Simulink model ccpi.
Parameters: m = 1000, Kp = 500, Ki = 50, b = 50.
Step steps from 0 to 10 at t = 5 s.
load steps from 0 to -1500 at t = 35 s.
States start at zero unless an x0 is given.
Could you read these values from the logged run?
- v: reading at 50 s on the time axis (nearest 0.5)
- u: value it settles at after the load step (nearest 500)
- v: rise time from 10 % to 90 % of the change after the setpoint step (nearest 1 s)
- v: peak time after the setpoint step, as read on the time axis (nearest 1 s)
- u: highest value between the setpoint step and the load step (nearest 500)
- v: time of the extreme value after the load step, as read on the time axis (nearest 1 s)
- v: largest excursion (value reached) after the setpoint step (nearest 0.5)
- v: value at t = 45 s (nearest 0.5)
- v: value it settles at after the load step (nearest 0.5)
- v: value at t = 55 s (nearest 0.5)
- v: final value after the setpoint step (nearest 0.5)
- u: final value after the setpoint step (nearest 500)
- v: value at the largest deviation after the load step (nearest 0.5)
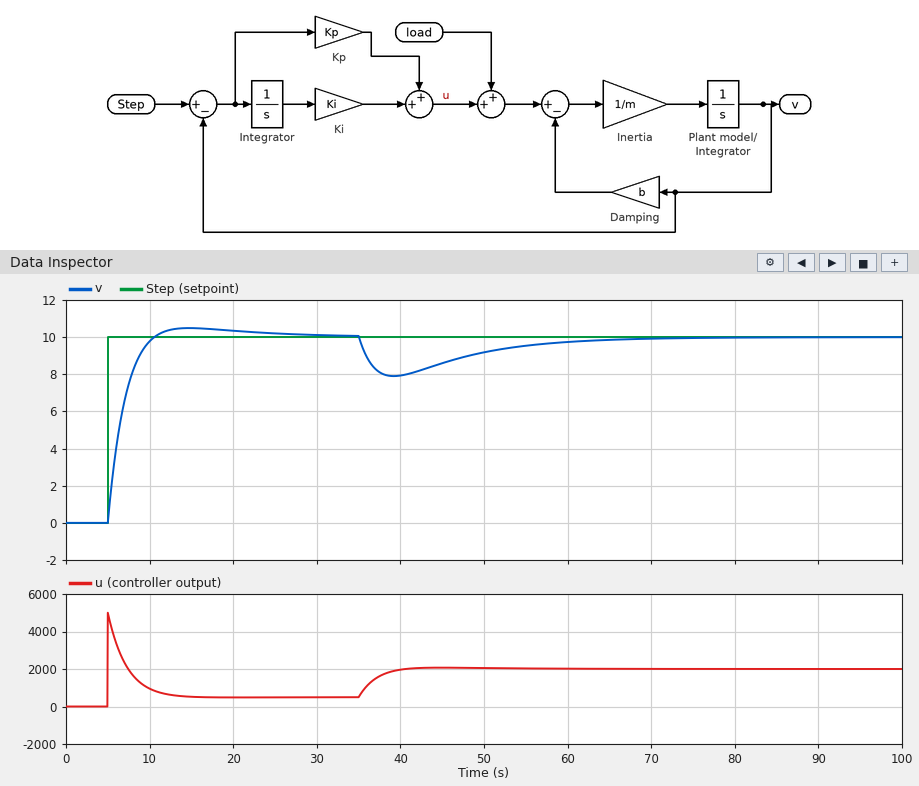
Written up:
9.0
2000
4 s
15 s
5000
39 s
10.5
8.5
10.0
9.5
10.0
500
8.0
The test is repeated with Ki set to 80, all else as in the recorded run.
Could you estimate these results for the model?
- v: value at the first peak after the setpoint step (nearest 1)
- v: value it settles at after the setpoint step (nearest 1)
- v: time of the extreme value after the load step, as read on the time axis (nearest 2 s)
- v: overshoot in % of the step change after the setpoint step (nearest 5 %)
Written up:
11
10
38 s
10 %
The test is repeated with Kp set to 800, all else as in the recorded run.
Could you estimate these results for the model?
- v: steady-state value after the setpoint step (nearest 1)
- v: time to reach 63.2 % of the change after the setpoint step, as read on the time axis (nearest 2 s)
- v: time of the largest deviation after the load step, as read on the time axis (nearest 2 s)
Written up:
10
6 s
38 s
